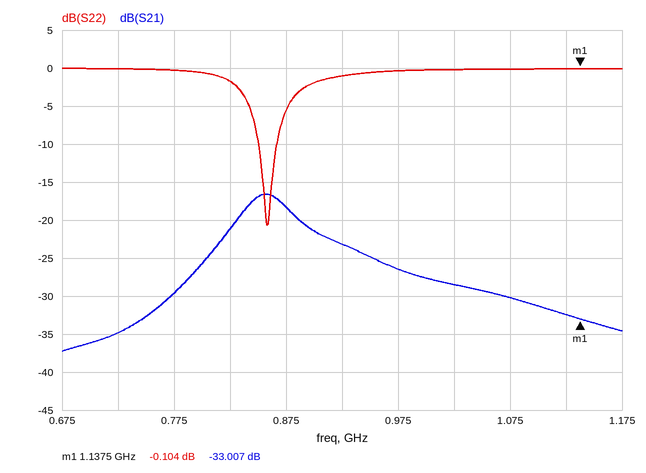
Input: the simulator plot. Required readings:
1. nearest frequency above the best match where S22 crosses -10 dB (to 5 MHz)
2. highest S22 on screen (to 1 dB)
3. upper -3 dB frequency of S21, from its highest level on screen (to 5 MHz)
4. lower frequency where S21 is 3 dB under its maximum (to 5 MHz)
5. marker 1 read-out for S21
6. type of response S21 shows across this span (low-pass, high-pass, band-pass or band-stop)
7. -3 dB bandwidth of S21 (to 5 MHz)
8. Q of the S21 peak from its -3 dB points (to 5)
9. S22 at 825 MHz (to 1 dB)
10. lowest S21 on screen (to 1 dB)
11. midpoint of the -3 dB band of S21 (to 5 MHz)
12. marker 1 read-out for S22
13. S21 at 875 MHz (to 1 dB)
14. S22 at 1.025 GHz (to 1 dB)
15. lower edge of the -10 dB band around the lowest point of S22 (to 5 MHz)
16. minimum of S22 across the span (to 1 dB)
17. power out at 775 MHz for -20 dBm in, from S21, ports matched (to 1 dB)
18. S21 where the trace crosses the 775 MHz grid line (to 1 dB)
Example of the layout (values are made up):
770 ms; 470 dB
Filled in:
865 MHz; 0 dB; 885 MHz; 835 MHz; -33.007 dB; band-pass; 50 MHz; 15; -2 dB; -37 dB; 860 MHz; -0.104 dB; -18 dB; 0 dB; 850 MHz; -21 dB; -50 dBm; -30 dB
